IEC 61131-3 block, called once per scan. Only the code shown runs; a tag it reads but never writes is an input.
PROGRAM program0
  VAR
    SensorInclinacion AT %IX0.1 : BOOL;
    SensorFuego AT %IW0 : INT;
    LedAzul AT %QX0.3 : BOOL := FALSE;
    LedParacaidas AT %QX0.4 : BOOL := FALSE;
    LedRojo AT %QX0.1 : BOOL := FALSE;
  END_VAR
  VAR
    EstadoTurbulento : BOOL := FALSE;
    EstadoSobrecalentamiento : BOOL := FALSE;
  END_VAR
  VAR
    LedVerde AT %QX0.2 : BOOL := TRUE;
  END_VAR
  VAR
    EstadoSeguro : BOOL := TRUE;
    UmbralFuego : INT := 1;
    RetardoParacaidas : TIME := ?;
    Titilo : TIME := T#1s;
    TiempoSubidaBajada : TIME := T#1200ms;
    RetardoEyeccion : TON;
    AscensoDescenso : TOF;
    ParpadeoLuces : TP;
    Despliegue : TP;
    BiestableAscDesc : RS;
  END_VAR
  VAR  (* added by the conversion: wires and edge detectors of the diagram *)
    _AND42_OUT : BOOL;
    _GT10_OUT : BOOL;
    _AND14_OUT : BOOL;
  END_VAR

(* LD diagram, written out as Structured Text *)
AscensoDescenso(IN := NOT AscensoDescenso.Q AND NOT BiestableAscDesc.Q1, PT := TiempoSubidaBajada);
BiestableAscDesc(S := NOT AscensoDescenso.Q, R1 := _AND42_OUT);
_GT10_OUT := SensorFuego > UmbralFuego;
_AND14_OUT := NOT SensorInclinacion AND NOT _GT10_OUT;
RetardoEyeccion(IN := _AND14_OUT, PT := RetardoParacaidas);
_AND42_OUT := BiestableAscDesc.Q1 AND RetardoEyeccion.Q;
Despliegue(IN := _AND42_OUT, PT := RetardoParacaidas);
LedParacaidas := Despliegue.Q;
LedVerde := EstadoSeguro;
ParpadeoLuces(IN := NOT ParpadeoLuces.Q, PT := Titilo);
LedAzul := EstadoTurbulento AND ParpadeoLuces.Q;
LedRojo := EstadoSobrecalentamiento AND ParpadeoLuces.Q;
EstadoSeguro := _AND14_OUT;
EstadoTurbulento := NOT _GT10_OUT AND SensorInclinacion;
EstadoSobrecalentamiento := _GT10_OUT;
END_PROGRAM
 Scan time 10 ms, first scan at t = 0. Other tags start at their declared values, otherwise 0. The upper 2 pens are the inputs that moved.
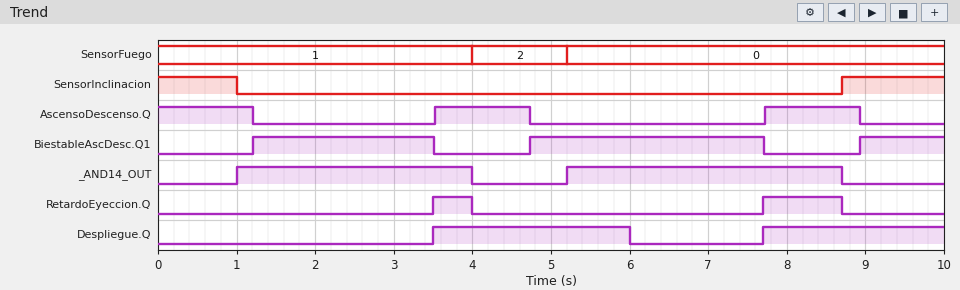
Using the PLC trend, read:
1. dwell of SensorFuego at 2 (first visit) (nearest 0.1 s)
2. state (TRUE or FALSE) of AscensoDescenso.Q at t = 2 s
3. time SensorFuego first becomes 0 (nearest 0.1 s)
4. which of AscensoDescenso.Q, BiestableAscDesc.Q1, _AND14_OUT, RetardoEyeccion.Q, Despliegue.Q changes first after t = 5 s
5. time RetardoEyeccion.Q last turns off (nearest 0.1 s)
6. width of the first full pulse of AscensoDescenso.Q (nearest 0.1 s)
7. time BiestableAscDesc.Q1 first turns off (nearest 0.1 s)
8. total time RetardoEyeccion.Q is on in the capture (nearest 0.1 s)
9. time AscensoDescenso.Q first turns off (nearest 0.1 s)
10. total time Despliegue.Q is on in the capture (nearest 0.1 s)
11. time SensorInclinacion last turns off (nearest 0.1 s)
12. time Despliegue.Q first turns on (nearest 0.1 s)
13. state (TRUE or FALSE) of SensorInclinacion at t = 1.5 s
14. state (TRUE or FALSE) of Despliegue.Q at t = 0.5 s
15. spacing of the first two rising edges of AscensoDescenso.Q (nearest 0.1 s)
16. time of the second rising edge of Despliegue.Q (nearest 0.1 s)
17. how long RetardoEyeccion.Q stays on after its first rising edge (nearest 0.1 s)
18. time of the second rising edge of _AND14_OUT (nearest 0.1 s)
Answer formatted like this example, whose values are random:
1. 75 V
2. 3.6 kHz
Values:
1. 1.2 s
2. FALSE
3. 5.2 s
4. _AND14_OUT
5. 8.7 s
6. 1.2 s
7. 3.5 s
8. 1.5 s
9. 1.2 s
10. 4.8 s
11. 1.0 s
12. 3.5 s
13. FALSE
14. FALSE
15. 4.2 s
16. 7.7 s
17. 0.5 s
18. 5.2 s
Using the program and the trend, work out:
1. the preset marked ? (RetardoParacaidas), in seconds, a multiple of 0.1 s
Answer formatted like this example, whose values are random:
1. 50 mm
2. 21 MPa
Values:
1. 2.5 s
